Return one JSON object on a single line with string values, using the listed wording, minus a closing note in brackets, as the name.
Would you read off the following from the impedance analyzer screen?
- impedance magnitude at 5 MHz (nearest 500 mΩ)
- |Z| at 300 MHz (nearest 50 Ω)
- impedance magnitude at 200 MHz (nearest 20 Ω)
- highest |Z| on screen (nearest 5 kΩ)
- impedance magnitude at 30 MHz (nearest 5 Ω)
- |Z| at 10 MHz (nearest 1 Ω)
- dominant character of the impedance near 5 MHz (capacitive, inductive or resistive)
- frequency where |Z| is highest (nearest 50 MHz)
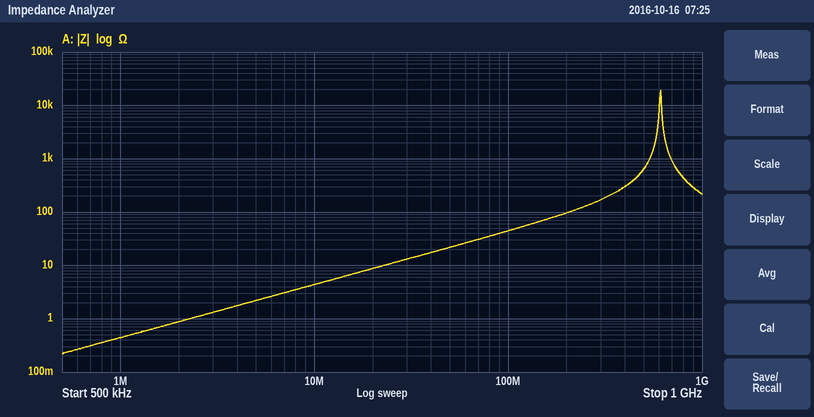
{"impedance magnitude at 5 MHz": "2.0 Ω", "|Z| at 300 MHz": "150 Ω", "impedance magnitude at 200 MHz": "100 Ω", "highest |Z| on screen": "20 kΩ", "impedance magnitude at 30 MHz": "15 Ω", "|Z| at 10 MHz": "4 Ω", "dominant character of the impedance near 5 MHz": "inductive", "frequency where |Z| is highest": "600 MHz"}
